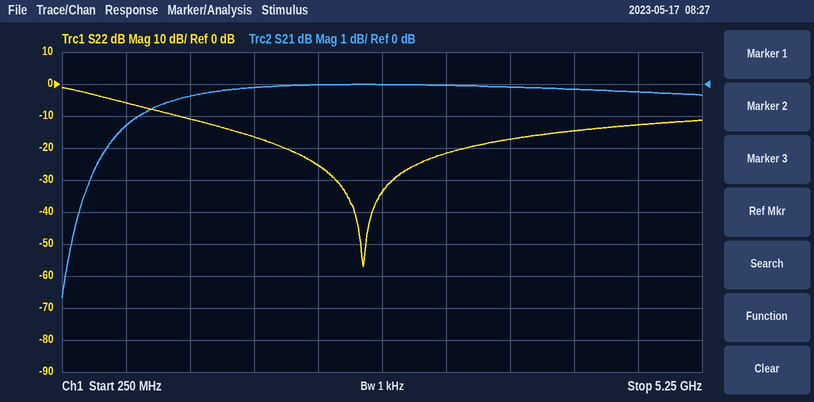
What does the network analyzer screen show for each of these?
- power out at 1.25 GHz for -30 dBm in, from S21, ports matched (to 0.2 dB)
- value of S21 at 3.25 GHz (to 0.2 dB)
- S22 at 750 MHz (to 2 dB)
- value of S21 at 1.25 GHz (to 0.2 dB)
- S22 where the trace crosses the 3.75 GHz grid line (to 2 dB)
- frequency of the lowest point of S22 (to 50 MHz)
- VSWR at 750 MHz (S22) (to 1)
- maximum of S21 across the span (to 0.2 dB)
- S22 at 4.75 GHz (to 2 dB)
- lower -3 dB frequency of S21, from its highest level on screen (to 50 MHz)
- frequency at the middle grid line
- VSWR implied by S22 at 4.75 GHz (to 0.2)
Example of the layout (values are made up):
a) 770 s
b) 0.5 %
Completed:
a) -30.4 dBm
b) 0.0 dB
c) -6 dB
d) -0.4 dB
e) -18 dB
f) 2.60 GHz
g) 3
h) 0.0 dB
i) -12 dB
j) 450 MHz
k) 2.75 GHz
l) 1.6
